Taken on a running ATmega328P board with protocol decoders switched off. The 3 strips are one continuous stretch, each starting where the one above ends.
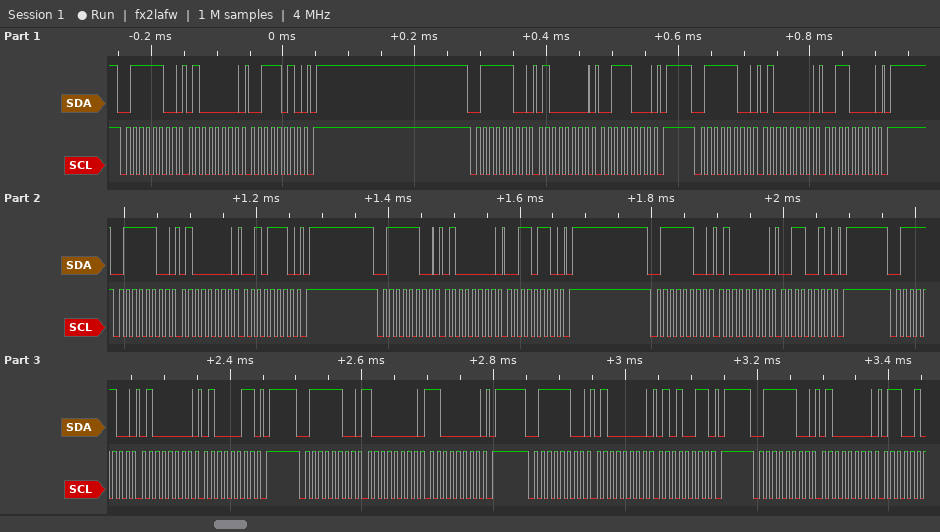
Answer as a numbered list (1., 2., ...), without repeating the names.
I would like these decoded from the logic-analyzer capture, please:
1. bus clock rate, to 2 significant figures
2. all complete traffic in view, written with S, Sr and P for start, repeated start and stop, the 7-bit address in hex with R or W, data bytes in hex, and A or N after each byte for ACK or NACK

1. 100 kHz
2. S 3EW A 40 A 3A A P S 3EW A 40 A 38 A P S 3EW A 40 A 30 A P S 3EW A 40 A 2E A P S 3EW A 40 A 36 A P S 3EW A 40 A 32 A P S 3EW A 40 A 43 A P S 3EW A 80 A C0 A P S 3EW A 40 A 53 A P S 3EW A 40 A
